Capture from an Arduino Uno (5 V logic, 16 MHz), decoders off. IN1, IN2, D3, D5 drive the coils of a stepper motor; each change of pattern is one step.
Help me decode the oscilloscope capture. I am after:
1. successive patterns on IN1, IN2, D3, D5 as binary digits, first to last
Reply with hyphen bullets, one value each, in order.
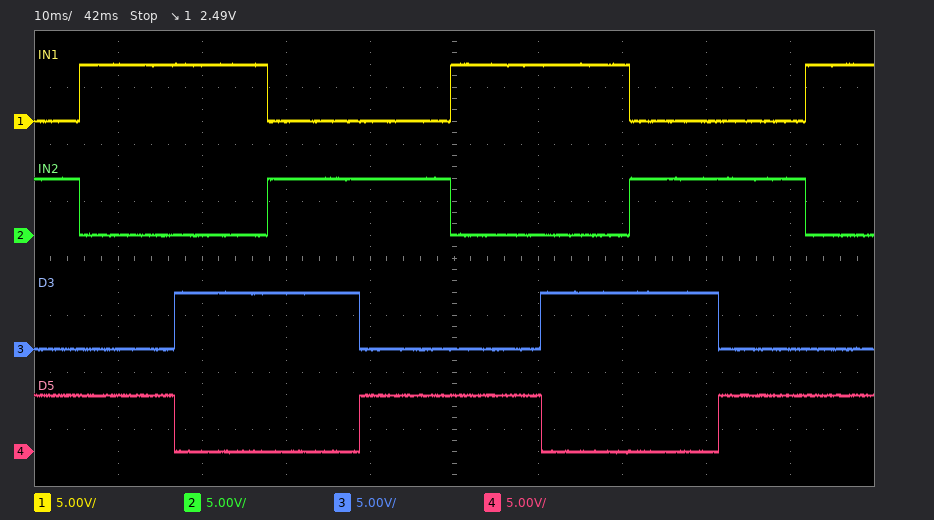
- 0101 1001 1010 0110 0101 1001 1010 0110 0101 1001
